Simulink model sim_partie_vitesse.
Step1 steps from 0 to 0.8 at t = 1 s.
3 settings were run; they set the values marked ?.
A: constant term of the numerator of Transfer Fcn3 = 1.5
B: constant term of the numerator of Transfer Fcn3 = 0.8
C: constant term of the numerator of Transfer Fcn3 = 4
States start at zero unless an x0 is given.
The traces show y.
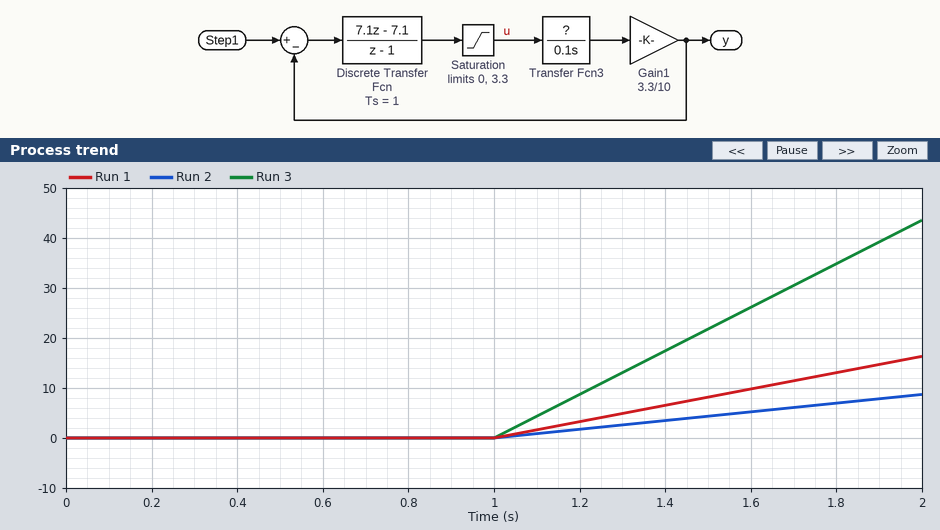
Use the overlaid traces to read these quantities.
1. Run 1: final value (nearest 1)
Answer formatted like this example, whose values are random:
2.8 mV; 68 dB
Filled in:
16
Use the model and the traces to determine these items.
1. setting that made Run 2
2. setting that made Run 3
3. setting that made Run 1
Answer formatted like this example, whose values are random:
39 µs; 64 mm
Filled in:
B; C; A
